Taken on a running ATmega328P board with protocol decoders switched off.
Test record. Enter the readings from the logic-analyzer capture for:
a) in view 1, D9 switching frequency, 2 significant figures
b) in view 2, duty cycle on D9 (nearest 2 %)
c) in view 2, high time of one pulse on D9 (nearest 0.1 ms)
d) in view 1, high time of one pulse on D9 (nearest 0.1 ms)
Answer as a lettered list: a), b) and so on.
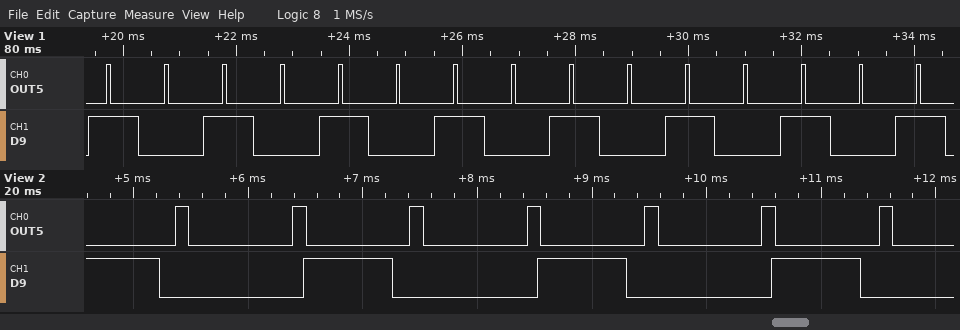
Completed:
a) 490 Hz
b) 38 %
c) 0.8 ms
d) 0.9 ms
